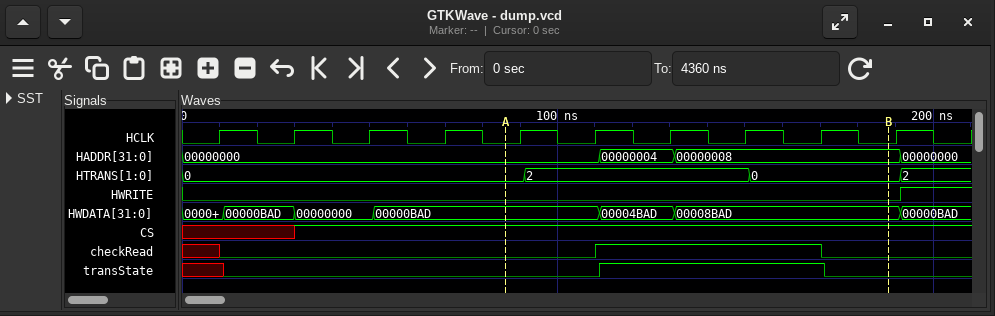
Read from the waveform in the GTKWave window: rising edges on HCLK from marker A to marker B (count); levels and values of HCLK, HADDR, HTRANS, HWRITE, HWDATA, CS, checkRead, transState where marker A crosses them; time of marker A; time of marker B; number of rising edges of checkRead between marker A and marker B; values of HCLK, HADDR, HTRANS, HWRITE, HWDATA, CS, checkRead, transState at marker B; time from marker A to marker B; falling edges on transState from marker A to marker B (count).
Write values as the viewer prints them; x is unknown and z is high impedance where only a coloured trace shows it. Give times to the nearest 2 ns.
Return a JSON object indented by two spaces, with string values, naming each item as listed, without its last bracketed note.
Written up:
{
  "rising edges on HCLK from marker A to marker B": "5",
  "levels and values of HCLK, HADDR, HTRANS, HWRITE, HWDATA, CS, checkRead, transState where marker A crosses them": "HCLK=0, HADDR=00000000, HTRANS=0, HWRITE=0, HWDATA=00000BAD, CS=1, checkRead=0, transState=0",
  "time of marker A": "86 ns",
  "time of marker B": "188 ns",
  "number of rising edges of checkRead between marker A and marker B": "1",
  "values of HCLK, HADDR, HTRANS, HWRITE, HWDATA, CS, checkRead, transState at marker B": "HCLK=0, HADDR=00000008, HTRANS=0, HWRITE=0, HWDATA=00008BAD, CS=1, checkRead=0, transState=0",
  "time from marker A to marker B": "102 ns",
  "falling edges on transState from marker A to marker B": "1"
}
